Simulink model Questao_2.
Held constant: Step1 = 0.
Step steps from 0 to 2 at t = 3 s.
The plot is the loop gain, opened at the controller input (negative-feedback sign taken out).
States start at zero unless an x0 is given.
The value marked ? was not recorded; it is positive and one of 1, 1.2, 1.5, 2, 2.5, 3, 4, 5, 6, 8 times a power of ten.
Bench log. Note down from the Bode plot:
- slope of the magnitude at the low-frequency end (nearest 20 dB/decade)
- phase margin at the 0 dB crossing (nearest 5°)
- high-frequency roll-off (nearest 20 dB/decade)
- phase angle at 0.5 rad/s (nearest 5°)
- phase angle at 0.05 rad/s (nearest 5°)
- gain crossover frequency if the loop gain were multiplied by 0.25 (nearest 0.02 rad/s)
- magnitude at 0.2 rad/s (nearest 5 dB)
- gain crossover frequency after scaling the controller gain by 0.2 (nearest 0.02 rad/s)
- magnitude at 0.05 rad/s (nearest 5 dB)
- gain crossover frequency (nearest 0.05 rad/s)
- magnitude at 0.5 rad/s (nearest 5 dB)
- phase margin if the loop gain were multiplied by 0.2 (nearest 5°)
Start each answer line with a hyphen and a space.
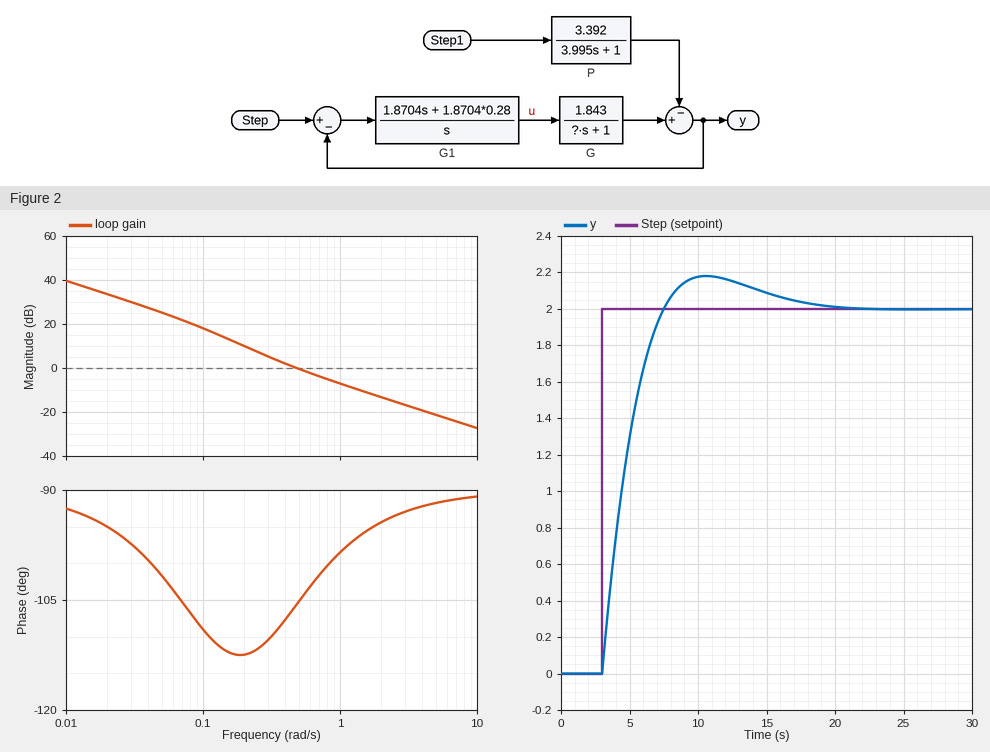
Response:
- -20 dB/decade
- 75°
- -20 dB/decade
- -105°
- -100°
- 0.16 rad/s
- 10 dB
- 0.14 rad/s
- 25 dB
- 0.50 rad/s
- 0 dB
- 70°
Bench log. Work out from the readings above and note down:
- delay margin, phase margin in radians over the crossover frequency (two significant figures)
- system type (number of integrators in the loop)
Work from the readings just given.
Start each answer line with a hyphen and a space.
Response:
- 2.6 s
- 1
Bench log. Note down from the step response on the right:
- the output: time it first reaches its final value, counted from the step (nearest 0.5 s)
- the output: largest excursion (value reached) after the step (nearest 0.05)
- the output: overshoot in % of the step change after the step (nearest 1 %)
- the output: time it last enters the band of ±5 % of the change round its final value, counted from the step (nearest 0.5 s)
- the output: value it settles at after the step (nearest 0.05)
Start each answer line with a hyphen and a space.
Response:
- 4.5 s
- 2.20
- 9 %
- 11.5 s
- 2.00
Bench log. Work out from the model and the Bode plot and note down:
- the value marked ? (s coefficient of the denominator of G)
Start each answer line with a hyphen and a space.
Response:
- 8
